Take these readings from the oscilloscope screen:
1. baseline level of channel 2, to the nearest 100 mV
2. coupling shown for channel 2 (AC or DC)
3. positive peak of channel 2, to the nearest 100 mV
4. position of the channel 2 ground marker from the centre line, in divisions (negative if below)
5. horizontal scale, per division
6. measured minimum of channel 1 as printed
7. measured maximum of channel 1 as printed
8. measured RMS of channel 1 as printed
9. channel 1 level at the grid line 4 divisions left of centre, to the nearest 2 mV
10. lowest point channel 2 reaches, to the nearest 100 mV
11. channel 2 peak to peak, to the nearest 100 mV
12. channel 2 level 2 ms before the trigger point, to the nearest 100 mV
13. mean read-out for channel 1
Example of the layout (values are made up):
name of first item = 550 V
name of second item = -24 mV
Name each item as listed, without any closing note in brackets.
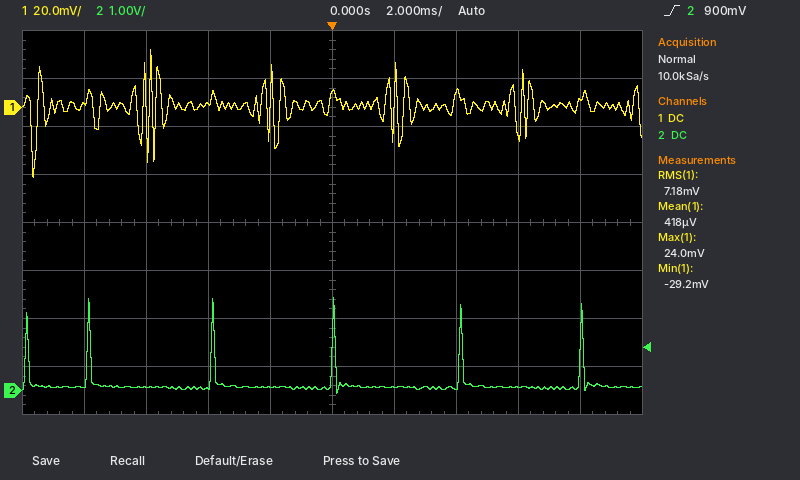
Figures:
baseline level of channel 2, to the nearest 100 mV = 100 mV
coupling shown for channel 2 = DC
positive peak of channel 2, to the nearest 100 mV = 1.9 V
position of the channel 2 ground marker from the centre line, in divisions = -3.5 div
horizontal scale, per division = 2 ms
measured minimum of channel 1 as printed = -29.2 mV
measured maximum of channel 1 as printed = 24.0 mV
measured RMS of channel 1 as printed = 7.18 mV
channel 1 level at the grid line 4 divisions left of centre, to the nearest 2 mV = 2 mV
lowest point channel 2 reaches, to the nearest 100 mV = -100 mV
channel 2 peak to peak, to the nearest 100 mV = 2.0 V
channel 2 level 2 ms before the trigger point, to the nearest 100 mV = 100 mV
mean read-out for channel 1 = 418 µV
